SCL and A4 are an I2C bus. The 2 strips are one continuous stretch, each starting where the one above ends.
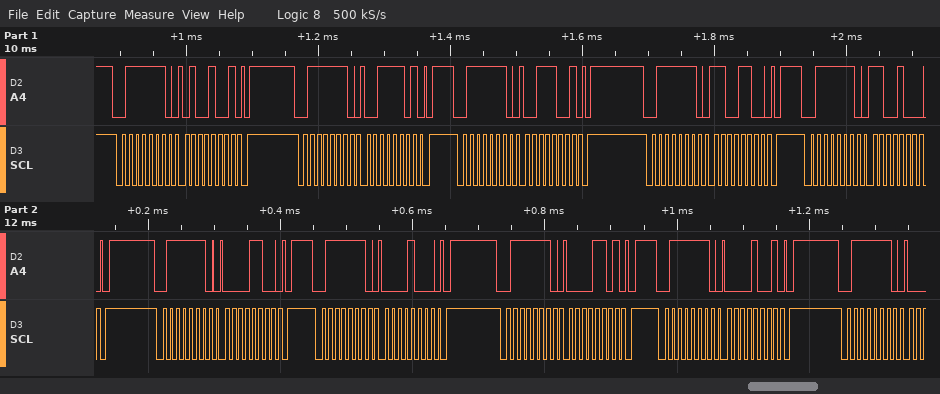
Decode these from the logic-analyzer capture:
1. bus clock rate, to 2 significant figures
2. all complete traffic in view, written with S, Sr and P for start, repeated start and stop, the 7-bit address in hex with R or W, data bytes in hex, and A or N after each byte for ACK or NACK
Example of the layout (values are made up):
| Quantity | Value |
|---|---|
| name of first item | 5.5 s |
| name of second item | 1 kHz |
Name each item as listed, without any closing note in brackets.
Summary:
| Quantity | Value |
|---|---|
| bus clock rate, to 2 significant figures | 100 kHz |
| all complete traffic in view, written with S, Sr and P for start, repeated start and stop, the 7-bit address in hex with R or W, data bytes in hex, and A or N after each byte for ACK or NACK | S 3FW A 49 A P S 3FW A 3D A P S 3FW A 39 A P S 3FW A CC A P S 3FW A C8 A P S 3FW A 0C A P S 3FW A 08 A P S 3FW A 0D A P S 3FW A 09 A P S 3FW A |
